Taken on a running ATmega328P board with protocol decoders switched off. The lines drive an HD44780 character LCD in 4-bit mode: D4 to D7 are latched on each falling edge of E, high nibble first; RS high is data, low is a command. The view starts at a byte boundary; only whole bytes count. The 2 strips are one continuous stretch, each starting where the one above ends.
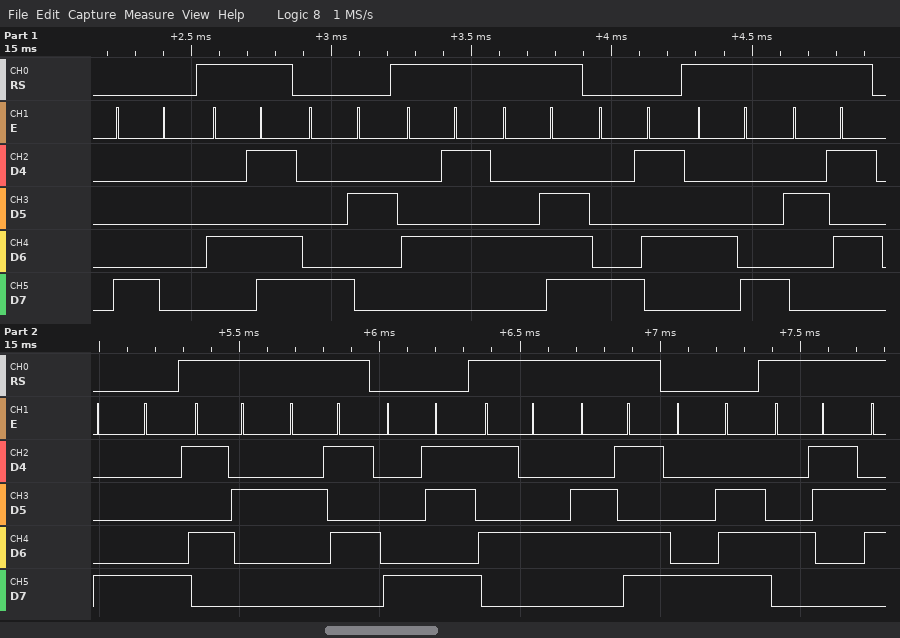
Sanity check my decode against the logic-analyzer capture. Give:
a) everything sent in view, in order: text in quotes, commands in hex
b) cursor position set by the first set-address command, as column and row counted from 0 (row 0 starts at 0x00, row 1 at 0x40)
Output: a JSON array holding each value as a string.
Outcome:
["0x80 \"M\" 0x82 \"EN\" 0x85 \"H%\" 0x88 \"R%\" 0x8B \"Tm\" 0x8E \"C\"", "column 0, row 0"]
